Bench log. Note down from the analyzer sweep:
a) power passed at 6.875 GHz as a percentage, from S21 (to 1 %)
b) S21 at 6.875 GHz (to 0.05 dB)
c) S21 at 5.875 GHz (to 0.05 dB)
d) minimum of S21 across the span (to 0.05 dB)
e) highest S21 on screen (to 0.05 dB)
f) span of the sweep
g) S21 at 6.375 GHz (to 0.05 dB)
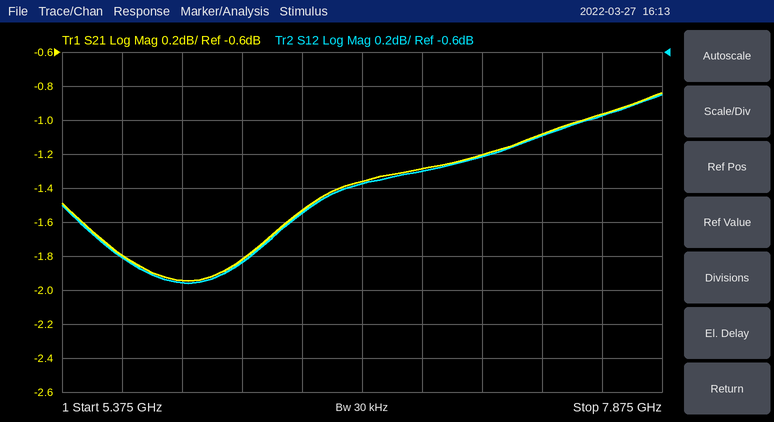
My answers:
74 %
-1.30 dB
-1.95 dB
-1.95 dB
-0.85 dB
2.5 GHz
-1.55 dB
